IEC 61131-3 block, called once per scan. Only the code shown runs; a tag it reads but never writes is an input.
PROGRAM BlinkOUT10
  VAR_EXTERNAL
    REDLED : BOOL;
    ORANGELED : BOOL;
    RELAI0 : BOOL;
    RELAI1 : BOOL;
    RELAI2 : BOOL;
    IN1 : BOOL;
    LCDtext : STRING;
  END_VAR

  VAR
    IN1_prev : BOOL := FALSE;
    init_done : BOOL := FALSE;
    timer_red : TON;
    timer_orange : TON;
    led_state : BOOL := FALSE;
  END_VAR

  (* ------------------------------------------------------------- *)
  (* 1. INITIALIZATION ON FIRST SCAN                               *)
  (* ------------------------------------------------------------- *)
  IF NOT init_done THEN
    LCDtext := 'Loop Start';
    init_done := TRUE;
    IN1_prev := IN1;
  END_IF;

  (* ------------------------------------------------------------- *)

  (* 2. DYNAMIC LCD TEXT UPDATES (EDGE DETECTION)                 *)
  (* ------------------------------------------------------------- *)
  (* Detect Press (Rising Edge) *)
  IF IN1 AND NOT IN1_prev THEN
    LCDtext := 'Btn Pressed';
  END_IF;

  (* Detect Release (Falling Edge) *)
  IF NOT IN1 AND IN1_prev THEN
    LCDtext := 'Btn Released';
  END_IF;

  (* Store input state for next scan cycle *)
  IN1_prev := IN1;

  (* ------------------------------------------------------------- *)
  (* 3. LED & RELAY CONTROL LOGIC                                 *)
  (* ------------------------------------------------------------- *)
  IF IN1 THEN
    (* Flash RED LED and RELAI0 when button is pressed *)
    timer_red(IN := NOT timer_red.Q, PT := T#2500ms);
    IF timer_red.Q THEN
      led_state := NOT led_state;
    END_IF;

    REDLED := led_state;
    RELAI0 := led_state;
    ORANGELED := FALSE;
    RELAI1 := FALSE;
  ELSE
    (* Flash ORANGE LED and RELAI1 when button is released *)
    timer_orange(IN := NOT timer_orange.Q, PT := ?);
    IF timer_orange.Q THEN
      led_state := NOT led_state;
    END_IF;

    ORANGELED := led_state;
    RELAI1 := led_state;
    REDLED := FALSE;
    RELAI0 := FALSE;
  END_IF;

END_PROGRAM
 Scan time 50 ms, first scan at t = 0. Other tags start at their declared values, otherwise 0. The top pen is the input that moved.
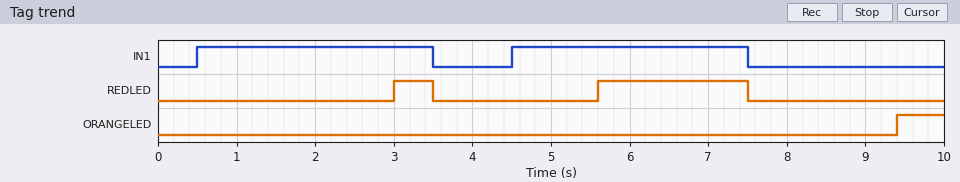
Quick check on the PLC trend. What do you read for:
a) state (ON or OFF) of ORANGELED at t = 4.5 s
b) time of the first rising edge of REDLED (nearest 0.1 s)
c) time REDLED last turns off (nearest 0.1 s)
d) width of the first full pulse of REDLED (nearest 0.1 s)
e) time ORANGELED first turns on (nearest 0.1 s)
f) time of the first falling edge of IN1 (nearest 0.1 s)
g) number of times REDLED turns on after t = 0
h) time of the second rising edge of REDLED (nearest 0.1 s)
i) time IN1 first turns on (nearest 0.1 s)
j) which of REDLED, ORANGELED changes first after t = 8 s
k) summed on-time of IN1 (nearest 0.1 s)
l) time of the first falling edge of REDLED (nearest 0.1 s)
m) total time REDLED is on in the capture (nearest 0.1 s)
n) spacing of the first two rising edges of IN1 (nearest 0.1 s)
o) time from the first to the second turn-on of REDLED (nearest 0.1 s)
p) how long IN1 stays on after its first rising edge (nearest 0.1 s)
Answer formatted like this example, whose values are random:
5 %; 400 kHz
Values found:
OFF; 3.0 s; 7.5 s; 0.5 s; 9.4 s; 3.5 s; 2; 5.6 s; 0.5 s; ORANGELED; 6.0 s; 3.5 s; 2.4 s; 4.0 s; 2.6 s; 3.0 s
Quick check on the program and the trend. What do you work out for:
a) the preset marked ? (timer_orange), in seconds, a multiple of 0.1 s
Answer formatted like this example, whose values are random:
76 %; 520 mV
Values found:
1.8 s
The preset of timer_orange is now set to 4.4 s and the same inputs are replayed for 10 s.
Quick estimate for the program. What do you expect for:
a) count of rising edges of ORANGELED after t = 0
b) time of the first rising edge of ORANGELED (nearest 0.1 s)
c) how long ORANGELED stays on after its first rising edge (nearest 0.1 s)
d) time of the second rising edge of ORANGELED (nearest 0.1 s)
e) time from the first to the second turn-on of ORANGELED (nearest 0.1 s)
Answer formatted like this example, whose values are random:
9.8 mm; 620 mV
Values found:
2; 3.5 s; 0.9 s; 7.5 s; 4.0 s
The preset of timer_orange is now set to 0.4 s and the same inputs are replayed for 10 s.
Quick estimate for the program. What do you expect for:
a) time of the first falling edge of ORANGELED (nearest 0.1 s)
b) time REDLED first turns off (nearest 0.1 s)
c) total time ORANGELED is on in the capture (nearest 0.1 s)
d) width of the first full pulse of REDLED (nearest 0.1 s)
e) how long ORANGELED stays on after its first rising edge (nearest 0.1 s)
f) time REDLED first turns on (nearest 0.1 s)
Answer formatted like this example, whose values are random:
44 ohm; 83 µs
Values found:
0.5 s; 3.0 s; 2.0 s; 2.5 s; 0.1 s; 0.5 s
